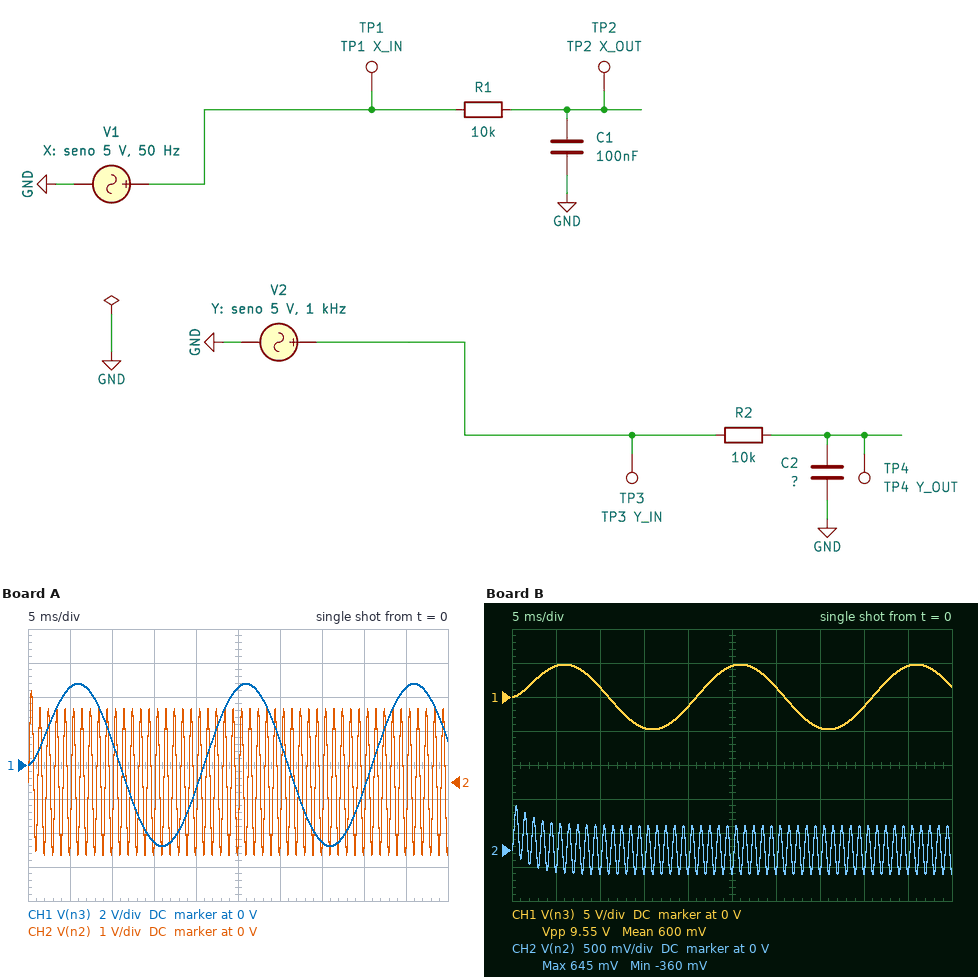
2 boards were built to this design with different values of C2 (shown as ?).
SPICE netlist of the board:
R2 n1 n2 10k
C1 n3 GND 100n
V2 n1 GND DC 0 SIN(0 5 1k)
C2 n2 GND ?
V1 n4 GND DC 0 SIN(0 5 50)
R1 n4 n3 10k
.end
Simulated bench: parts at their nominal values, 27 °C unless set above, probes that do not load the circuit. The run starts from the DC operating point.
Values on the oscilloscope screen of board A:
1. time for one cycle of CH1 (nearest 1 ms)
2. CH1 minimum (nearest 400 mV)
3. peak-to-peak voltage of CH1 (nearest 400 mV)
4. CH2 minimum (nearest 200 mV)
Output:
20 ms
-4.8 V
9.6 V
-2.2 V
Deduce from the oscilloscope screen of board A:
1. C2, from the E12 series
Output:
33 nF
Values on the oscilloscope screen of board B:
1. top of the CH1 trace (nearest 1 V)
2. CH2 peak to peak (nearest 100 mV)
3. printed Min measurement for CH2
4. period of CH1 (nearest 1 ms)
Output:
5 V
1.0 V
-360 mV
20 ms
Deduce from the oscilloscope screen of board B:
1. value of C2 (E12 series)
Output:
220 nF
